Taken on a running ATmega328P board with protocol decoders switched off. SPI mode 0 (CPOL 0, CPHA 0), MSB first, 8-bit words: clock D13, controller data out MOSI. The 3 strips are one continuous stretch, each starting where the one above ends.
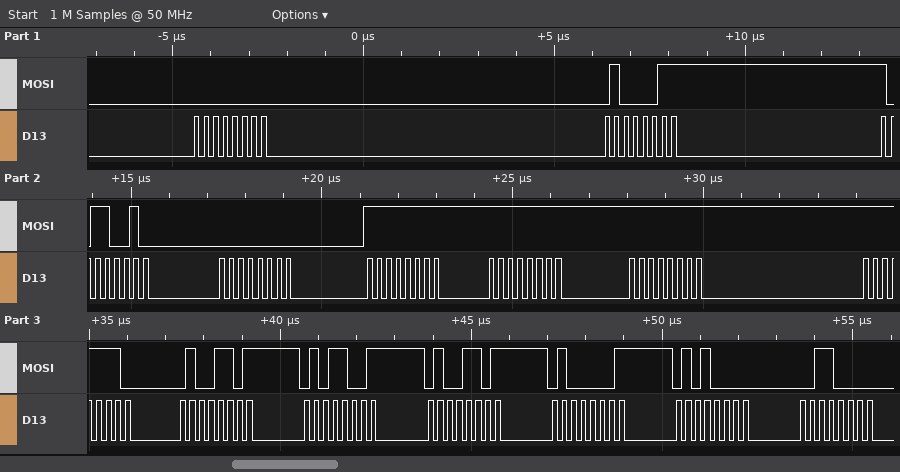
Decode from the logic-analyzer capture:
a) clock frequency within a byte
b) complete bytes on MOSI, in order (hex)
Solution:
4 MHz
0x00 0x43 0xB2 0x00 0xFF 0xFF 0xFF 0xFE 0x4D 0x59 0x4D 0x41 0x50 0x30
